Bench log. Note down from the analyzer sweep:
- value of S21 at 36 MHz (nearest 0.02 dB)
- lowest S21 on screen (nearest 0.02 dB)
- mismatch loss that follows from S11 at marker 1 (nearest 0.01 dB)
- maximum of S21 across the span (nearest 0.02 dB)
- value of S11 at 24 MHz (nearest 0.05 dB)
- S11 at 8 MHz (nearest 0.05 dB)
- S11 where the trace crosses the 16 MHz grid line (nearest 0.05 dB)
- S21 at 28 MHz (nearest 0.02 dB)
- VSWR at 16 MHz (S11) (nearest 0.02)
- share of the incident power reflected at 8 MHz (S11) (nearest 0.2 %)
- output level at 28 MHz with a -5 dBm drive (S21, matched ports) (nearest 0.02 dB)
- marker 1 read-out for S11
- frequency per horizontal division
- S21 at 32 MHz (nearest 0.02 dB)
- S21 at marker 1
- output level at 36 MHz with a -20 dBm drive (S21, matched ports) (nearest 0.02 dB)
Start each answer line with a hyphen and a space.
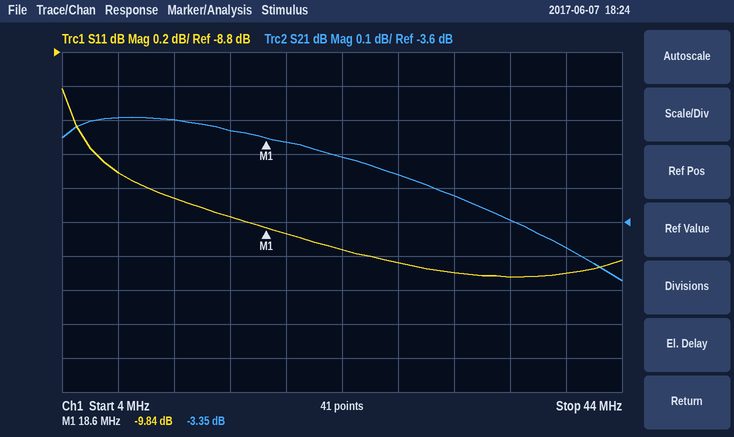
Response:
- -3.60 dB
- -3.78 dB
- 0.48 dB
- -3.30 dB
- -9.95 dB
- -9.50 dB
- -9.75 dB
- -3.46 dB
- 1.96
- 11.2 %
- -8.46 dBm
- -9.84 dB
- 4 MHz
- -3.52 dB
- -3.35 dB
- -23.60 dBm
